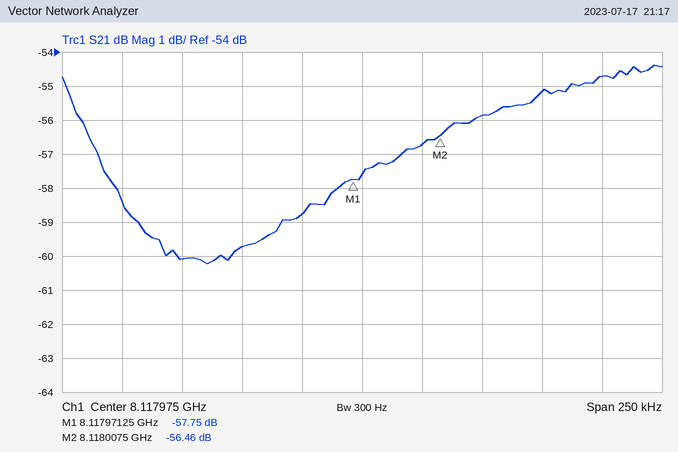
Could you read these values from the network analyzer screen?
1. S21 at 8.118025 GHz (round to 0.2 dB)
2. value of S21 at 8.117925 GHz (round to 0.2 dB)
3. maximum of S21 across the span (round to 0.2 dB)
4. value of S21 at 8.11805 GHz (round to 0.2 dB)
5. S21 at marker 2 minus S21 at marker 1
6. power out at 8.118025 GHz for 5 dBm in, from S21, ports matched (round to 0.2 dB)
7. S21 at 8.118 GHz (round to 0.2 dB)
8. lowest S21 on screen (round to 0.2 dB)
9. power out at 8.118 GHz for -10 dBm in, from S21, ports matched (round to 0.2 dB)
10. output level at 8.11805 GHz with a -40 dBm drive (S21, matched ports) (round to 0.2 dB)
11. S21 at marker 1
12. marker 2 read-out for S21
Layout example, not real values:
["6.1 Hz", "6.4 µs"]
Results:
["-55.8 dB", "-59.8 dB", "-54.4 dB", "-55.2 dB", "1.29 dB", "-50.8 dBm", "-56.8 dB", "-60.2 dB", "-66.8 dBm", "-95.2 dBm", "-57.75 dB", "-56.46 dB"]
